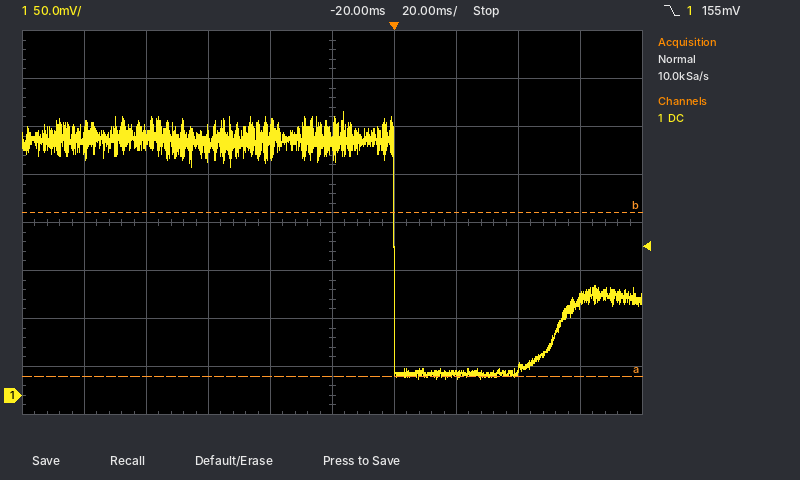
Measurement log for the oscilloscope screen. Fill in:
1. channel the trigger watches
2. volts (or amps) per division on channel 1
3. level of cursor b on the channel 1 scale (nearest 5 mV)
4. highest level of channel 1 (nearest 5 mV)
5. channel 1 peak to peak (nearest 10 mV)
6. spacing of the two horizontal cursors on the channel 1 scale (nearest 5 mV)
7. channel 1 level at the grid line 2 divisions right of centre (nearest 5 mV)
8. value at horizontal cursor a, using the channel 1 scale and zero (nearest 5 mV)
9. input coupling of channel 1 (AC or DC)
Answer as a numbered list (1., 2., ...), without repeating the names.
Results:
1. channel 1
2. 50 mV
3. 190 mV
4. 295 mV
5. 280 mV
6. 170 mV
7. 20 mV
8. 20 mV
9. DC
